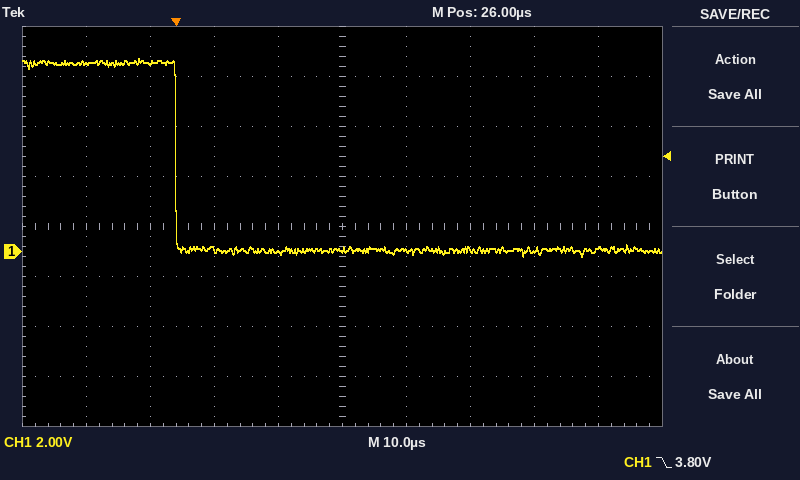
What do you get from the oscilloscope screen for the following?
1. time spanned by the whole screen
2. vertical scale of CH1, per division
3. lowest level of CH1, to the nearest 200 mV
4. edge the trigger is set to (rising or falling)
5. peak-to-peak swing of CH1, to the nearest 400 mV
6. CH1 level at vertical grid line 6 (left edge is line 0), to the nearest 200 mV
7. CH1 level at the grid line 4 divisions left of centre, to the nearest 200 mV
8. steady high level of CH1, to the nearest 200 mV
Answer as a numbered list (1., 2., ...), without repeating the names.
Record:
1. 100 µs
2. 2 V
3. -200 mV
4. falling
5. 8.0 V
6. 0.0 V
7. 7.6 V
8. 7.6 V
